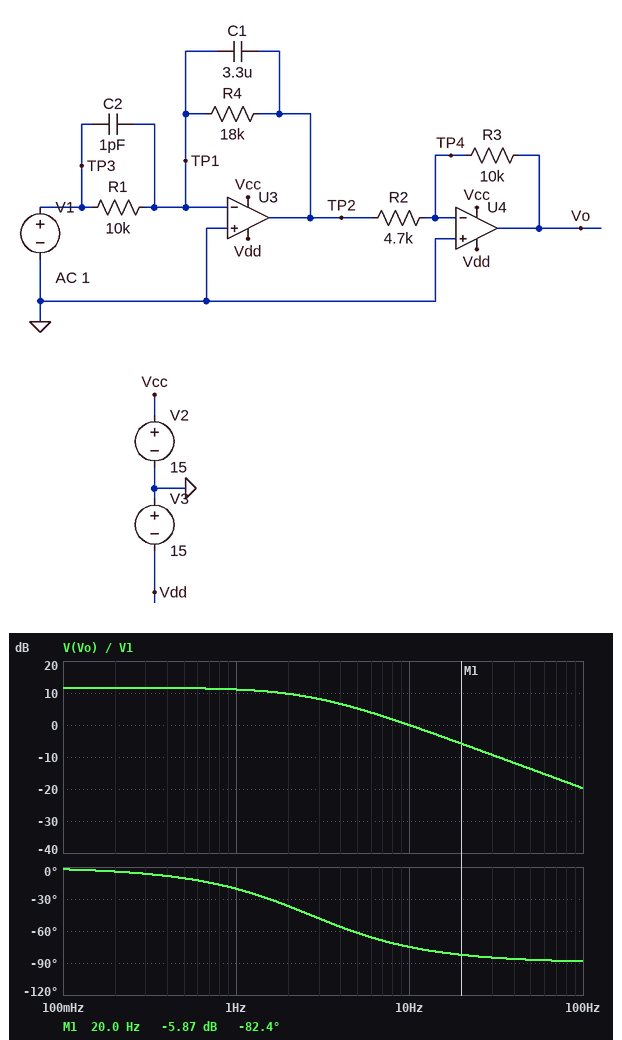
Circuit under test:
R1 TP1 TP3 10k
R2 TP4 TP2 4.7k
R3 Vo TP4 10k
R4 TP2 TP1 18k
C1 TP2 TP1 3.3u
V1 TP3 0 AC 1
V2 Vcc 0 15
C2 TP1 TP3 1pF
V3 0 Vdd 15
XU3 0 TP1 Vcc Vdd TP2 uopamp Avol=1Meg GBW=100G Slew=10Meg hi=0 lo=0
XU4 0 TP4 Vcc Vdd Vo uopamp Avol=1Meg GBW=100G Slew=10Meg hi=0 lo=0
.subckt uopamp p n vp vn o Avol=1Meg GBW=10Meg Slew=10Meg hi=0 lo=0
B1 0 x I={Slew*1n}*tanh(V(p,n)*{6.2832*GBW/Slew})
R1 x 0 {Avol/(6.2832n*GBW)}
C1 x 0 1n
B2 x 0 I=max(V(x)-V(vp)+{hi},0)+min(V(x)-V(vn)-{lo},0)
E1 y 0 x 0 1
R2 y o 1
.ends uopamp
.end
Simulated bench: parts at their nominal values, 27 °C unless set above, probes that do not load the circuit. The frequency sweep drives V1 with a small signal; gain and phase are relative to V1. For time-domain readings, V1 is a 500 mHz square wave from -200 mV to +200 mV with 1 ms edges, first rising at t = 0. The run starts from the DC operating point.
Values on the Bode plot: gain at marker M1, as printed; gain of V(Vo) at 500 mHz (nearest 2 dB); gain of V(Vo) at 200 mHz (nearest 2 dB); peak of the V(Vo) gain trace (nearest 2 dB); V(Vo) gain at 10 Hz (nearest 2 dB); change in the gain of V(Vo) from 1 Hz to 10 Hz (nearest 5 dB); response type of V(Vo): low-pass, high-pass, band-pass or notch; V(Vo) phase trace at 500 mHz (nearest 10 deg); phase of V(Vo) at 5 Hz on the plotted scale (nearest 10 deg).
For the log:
-5.87 dB
12 dB
12 dB
12 dB
0 dB
-10 dB
low-pass
-10 deg
-60 deg
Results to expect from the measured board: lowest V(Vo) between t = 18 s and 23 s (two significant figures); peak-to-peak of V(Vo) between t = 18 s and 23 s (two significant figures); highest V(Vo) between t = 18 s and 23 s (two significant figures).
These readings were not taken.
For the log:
-770 mV
1.5 V
770 mV
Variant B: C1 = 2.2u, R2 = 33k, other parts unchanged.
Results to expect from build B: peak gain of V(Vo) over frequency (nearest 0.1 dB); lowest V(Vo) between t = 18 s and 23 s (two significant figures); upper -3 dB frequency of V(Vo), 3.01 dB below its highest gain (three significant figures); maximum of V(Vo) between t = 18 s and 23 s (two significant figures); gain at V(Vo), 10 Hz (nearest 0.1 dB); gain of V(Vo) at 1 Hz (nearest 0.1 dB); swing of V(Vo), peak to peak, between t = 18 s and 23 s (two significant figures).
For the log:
-5.3 dB
-110 mV
4.02 Hz
110 mV
-13.8 dB
-5.5 dB
220 mV
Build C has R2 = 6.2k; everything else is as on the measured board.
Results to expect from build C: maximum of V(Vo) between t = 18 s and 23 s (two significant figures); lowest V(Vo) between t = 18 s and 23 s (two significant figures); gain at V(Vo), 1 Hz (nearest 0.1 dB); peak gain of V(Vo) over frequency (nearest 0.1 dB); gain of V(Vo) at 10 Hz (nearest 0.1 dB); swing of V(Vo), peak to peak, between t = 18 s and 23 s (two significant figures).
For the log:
580 mV
-580 mV
8.7 dB
9.3 dB
-2.5 dB
1.2 V
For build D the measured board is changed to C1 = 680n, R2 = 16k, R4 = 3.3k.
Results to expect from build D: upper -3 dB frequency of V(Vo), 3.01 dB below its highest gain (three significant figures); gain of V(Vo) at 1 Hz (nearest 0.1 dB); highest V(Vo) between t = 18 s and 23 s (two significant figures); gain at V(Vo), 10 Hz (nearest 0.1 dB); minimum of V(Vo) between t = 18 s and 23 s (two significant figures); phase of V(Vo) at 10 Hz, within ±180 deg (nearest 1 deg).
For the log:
70.9 Hz
-13.7 dB
41 mV
-13.8 dB
-41 mV
-8 deg
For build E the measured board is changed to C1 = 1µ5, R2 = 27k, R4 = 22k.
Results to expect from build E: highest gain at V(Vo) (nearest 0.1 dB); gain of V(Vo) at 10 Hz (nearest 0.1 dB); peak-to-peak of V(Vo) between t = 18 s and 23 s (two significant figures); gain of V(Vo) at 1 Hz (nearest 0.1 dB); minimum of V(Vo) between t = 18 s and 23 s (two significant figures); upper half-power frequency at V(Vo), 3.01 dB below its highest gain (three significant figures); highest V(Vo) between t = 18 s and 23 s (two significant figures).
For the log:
-1.8 dB
-9.0 dB
330 mV
-2.0 dB
-160 mV
4.82 Hz
160 mV
